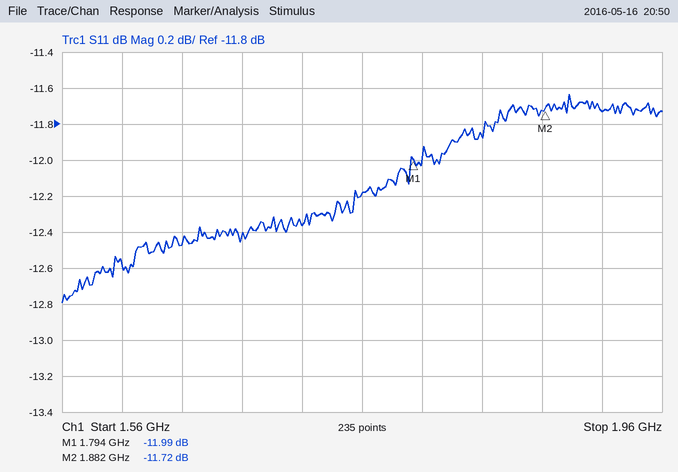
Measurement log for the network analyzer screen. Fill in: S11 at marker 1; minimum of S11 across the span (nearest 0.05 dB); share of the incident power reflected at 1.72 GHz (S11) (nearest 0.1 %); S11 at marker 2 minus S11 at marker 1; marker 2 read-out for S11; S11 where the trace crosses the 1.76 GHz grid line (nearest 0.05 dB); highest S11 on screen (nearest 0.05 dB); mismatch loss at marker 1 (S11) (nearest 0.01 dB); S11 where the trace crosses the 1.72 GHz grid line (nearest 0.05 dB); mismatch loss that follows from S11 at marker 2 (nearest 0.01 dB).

-11.99 dB
-12.80 dB
5.8 %
0.27 dB
-11.72 dB
-12.20 dB
-11.65 dB
0.28 dB
-12.35 dB
0.30 dB
